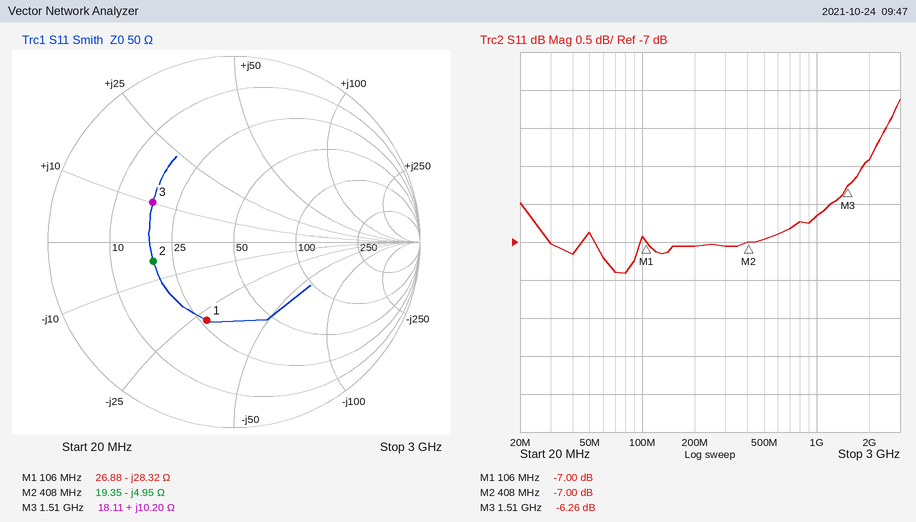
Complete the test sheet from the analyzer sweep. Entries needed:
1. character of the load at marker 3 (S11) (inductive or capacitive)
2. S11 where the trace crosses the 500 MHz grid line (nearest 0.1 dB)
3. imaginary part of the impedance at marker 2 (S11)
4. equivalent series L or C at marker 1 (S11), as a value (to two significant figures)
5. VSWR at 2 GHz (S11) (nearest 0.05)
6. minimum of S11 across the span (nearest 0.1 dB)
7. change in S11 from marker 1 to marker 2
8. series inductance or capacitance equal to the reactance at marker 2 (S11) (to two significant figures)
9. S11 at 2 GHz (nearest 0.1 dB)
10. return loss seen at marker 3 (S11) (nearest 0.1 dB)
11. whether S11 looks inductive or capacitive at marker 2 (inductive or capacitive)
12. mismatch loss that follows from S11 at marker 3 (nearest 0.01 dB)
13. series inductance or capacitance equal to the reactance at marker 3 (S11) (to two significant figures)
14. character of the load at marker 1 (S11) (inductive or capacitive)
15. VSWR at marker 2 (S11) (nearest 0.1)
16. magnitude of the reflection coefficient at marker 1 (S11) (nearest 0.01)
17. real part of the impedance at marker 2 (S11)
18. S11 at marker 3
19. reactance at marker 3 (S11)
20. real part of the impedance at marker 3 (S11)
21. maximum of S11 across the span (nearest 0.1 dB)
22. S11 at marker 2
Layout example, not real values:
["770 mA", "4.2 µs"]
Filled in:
["inductive", "-7.0 dB", "-4.95 Ω", "53 pF", "3.05", "-7.4 dB", "0.00 dB", "79 pF", "-5.9 dB", "6.3 dB", "capacitive", "1.17 dB", "1.1 nH", "capacitive", "2.6", "0.45", "19.35 Ω", "-6.26 dB", "+10.20 Ω", "18.11 Ω", "-5.1 dB", "-7.00 dB"]
